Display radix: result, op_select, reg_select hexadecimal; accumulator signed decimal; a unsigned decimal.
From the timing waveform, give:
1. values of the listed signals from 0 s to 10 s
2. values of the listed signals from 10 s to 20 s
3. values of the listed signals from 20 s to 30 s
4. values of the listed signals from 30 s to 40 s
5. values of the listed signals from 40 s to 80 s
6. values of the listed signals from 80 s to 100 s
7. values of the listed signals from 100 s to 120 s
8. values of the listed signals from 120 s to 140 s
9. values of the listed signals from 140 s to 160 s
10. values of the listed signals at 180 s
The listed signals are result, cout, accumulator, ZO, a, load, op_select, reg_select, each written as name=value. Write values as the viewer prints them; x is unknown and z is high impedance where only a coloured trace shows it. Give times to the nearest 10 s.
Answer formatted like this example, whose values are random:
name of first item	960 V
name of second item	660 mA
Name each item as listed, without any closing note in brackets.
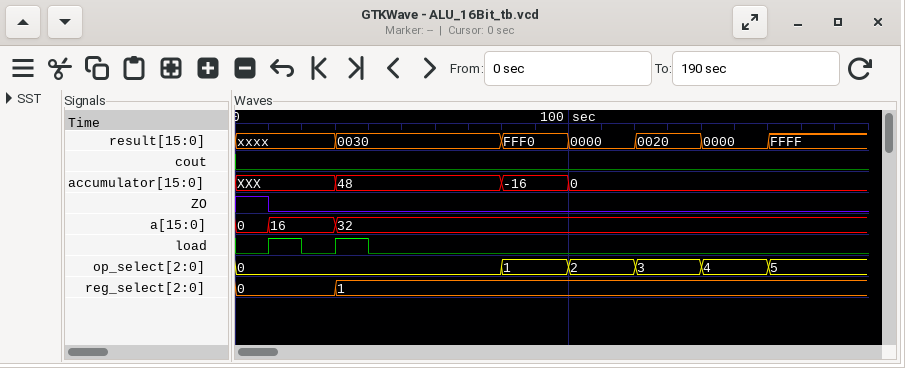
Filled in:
values of the listed signals from 0 s to 10 s	result=xxxx, cout=0, accumulator=XXX, ZO=1, a=0, load=0, op_select=0, reg_select=0
values of the listed signals from 10 s to 20 s	result=xxxx, cout=0, accumulator=XXX, ZO=0, a=16, load=1, op_select=0, reg_select=0
values of the listed signals from 20 s to 30 s	result=xxxx, cout=0, accumulator=XXX, ZO=0, a=16, load=0, op_select=0, reg_select=0
values of the listed signals from 30 s to 40 s	result=0030, cout=0, accumulator=48, ZO=0, a=32, load=1, op_select=0, reg_select=1
values of the listed signals from 40 s to 80 s	result=0030, cout=0, accumulator=48, ZO=0, a=32, load=0, op_select=0, reg_select=1
values of the listed signals from 80 s to 100 s	result=FFF0, cout=0, accumulator=-16, ZO=0, a=32, load=0, op_select=1, reg_select=1
values of the listed signals from 100 s to 120 s	result=0000, cout=0, accumulator=0, ZO=0, a=32, load=0, op_select=2, reg_select=1
values of the listed signals from 120 s to 140 s	result=0020, cout=0, accumulator=0, ZO=0, a=32, load=0, op_select=3, reg_select=1
values of the listed signals from 140 s to 160 s	result=0000, cout=0, accumulator=0, ZO=0, a=32, load=0, op_select=4, reg_select=1
values of the listed signals at 180 s	result=FFFF, cout=0, accumulator=0, ZO=0, a=32, load=0, op_select=5, reg_select=1
